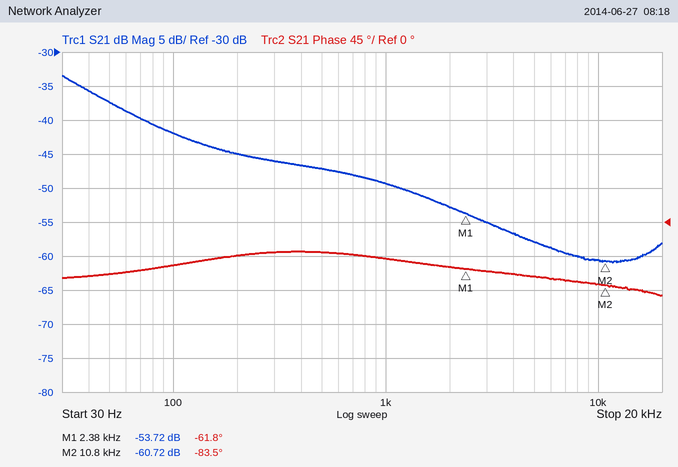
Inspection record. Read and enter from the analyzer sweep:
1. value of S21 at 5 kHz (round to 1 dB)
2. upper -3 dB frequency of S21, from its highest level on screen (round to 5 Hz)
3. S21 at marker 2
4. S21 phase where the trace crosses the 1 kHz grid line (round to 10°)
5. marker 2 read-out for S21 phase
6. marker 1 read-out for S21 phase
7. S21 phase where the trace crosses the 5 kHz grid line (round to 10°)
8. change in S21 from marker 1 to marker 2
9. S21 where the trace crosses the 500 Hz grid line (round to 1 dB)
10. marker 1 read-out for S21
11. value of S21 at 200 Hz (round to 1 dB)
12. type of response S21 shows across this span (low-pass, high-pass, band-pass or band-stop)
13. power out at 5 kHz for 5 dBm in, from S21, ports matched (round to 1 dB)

-58 dB
45 Hz
-60.72 dB
-50°
-83.5°
-61.8°
-70°
-7.00 dB
-47 dB
-53.72 dB
-45 dB
low-pass
-53 dBm
